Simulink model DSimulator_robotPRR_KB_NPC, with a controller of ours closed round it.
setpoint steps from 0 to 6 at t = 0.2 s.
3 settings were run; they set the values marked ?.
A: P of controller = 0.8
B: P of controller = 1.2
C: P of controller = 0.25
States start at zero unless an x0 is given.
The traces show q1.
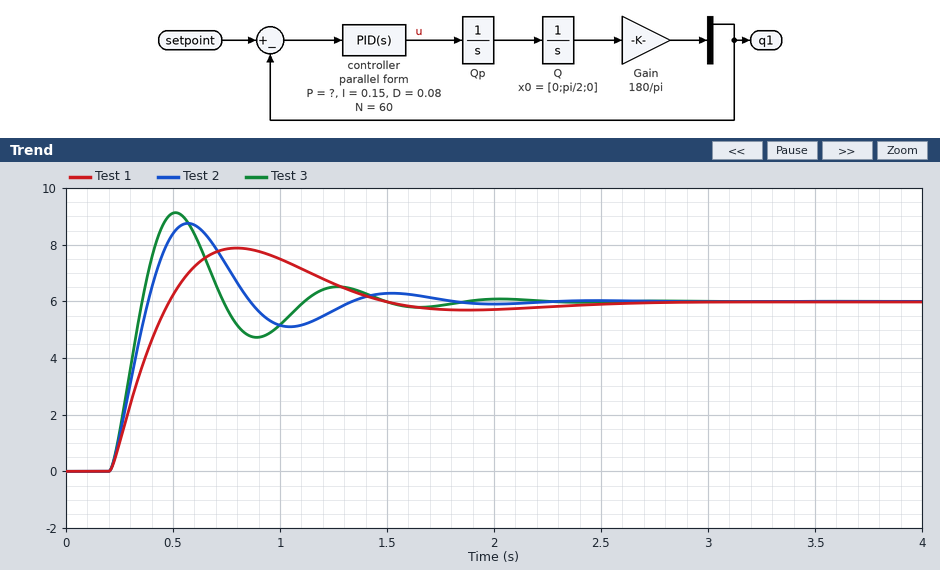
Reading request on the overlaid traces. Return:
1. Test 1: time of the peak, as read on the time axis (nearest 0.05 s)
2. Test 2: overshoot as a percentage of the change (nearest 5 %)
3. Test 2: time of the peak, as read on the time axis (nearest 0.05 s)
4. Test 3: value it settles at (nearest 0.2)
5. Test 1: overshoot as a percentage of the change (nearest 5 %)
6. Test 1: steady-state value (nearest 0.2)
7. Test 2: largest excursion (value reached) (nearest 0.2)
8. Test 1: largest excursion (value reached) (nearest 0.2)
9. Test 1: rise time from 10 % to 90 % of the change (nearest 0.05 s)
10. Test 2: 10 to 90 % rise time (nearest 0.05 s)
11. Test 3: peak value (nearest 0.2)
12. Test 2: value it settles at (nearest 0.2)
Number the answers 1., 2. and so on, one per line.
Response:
1. 0.80 s
2. 45 %
3. 0.55 s
4. 6.0
5. 30 %
6. 6.0
7. 8.8
8. 7.8
9. 0.20 s
10. 0.15 s
11. 9.2
12. 6.0
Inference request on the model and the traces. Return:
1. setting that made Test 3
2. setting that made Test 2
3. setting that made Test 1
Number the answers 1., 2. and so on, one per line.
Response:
1. B
2. A
3. C
